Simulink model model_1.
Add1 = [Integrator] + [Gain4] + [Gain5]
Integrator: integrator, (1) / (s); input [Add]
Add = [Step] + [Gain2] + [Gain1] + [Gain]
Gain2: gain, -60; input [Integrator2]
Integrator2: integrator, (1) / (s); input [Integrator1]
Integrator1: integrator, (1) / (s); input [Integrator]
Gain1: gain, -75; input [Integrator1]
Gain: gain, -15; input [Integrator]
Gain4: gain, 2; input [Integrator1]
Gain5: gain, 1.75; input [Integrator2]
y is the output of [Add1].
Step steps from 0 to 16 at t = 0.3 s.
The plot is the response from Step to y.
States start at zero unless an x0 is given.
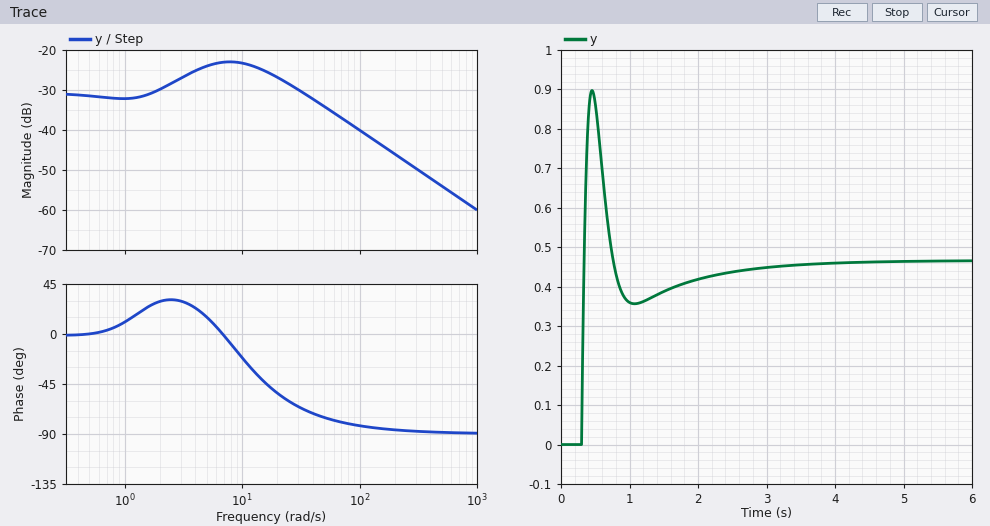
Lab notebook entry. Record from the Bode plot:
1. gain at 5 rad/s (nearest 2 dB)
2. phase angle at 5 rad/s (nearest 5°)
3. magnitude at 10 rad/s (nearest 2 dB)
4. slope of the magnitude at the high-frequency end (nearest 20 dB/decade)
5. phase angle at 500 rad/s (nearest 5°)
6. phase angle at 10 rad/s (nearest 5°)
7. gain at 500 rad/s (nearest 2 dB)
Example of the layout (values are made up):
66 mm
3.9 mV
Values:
-24 dB
15°
-24 dB
-20 dB/decade
-90°
-20°
-54 dB
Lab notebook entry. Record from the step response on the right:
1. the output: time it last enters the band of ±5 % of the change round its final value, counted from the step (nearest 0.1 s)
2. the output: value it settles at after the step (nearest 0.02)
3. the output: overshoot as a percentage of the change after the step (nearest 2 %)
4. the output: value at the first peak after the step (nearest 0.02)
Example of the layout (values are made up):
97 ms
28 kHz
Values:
2.4 s
0.46
92 %
0.90
